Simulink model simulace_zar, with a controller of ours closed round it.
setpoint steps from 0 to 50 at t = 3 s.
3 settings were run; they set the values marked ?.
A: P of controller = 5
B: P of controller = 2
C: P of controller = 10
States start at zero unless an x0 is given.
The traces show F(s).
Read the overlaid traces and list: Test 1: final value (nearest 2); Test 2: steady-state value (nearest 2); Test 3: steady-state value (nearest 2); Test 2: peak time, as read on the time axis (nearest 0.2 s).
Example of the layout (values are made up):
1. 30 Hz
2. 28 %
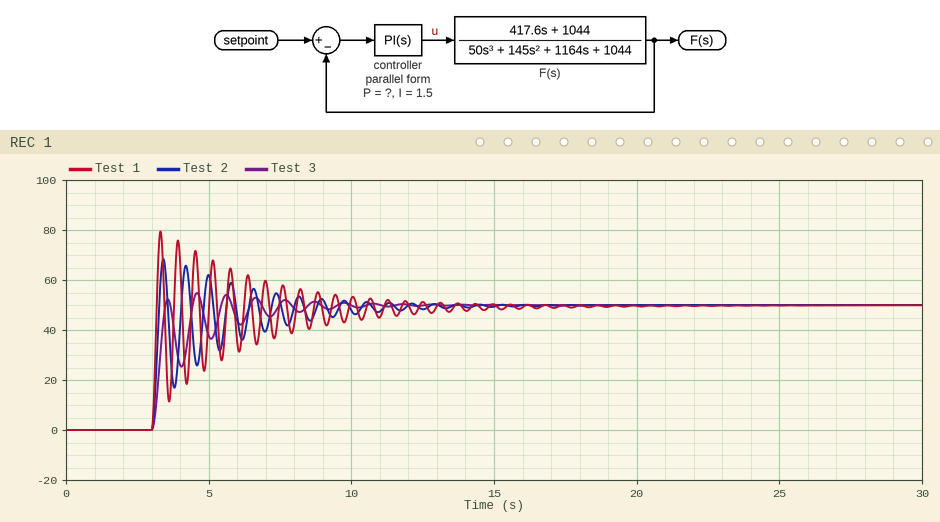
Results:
1. 50
2. 50
3. 50
4. 3.4 s
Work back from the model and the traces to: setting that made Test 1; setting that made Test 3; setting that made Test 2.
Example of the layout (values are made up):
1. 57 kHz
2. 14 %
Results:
1. C
2. B
3. A
